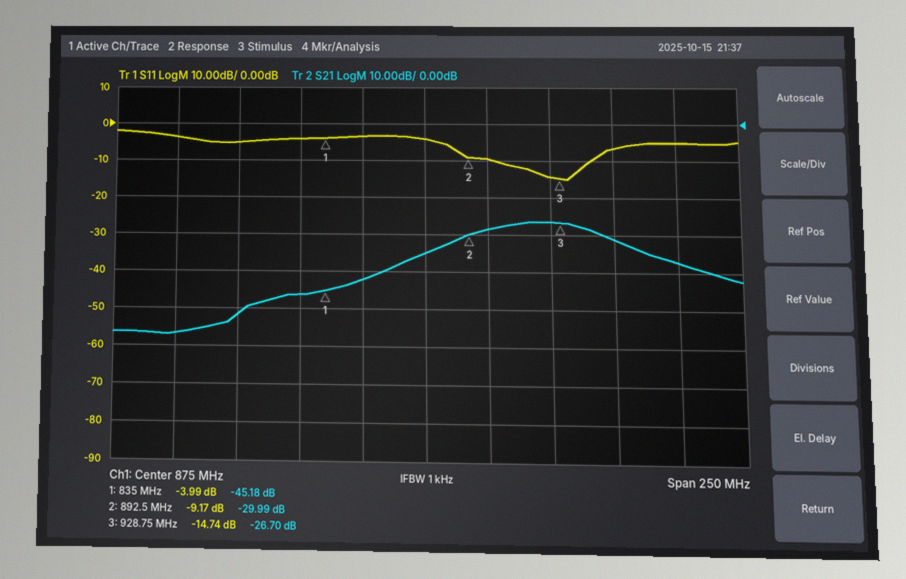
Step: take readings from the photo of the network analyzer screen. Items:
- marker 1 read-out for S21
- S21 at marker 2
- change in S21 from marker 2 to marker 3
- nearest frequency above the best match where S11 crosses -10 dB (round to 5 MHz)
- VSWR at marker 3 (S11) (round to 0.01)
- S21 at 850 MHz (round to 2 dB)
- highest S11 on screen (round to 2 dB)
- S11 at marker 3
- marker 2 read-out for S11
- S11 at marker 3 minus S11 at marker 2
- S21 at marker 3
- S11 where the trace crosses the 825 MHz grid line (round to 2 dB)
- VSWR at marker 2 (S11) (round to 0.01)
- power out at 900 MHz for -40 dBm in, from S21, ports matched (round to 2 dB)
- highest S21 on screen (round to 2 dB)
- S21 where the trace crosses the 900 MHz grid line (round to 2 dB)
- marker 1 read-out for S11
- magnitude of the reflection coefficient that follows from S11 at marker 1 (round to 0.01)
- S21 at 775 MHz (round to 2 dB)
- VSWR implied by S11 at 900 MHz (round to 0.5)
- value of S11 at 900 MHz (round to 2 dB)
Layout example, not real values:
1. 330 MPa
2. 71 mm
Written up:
1. -45.18 dB
2. -29.99 dB
3. 3.29 dB
4. 940 MHz
5. 1.45
6. -42 dB
7. -2 dB
8. -14.74 dB
9. -9.17 dB
10. -5.57 dB
11. -26.70 dB
12. -4 dB
13. 2.07
14. -68 dBm
15. -26 dB
16. -28 dB
17. -3.99 dB
18. 0.63
19. -56 dB
20. 2.0
21. -10 dB
